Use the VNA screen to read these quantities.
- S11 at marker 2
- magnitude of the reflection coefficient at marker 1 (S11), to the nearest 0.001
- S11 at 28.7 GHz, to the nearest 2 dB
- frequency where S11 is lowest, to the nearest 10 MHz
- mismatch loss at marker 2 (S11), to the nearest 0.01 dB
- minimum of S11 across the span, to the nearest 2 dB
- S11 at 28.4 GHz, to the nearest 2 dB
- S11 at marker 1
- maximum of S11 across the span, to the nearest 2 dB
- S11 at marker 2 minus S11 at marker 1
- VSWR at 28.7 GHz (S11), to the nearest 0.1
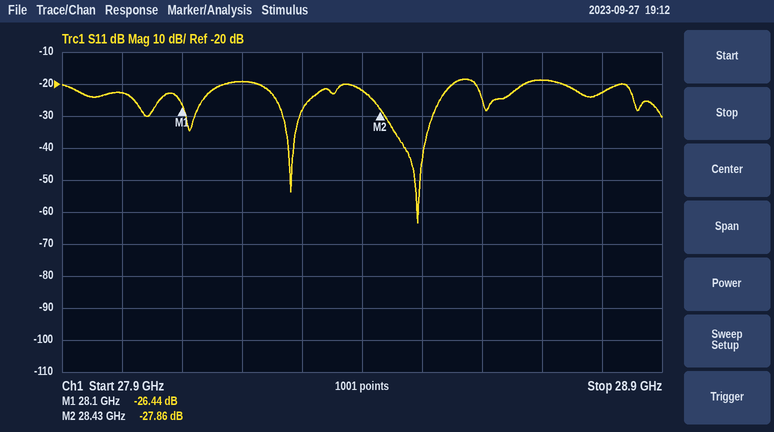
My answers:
-27.86 dB
0.048
-18 dB
28.49 GHz
0.01 dB
-64 dB
-22 dB
-26.44 dB
-18 dB
-1.42 dB
1.3
